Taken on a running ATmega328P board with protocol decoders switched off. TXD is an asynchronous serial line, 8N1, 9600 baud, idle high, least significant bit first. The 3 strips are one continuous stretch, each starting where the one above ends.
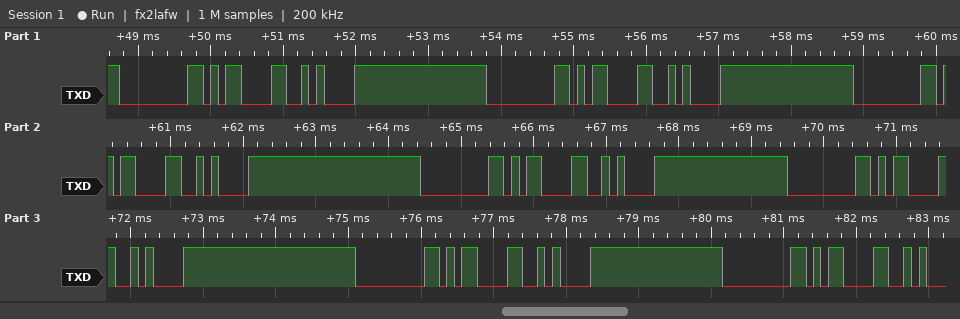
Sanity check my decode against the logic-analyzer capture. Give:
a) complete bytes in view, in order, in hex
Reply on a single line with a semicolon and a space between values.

00 0D 0A 00 0D 0A 00 0D 0A 00 0D 0A 00 0D 0A 00 0D 0A 00 0D
